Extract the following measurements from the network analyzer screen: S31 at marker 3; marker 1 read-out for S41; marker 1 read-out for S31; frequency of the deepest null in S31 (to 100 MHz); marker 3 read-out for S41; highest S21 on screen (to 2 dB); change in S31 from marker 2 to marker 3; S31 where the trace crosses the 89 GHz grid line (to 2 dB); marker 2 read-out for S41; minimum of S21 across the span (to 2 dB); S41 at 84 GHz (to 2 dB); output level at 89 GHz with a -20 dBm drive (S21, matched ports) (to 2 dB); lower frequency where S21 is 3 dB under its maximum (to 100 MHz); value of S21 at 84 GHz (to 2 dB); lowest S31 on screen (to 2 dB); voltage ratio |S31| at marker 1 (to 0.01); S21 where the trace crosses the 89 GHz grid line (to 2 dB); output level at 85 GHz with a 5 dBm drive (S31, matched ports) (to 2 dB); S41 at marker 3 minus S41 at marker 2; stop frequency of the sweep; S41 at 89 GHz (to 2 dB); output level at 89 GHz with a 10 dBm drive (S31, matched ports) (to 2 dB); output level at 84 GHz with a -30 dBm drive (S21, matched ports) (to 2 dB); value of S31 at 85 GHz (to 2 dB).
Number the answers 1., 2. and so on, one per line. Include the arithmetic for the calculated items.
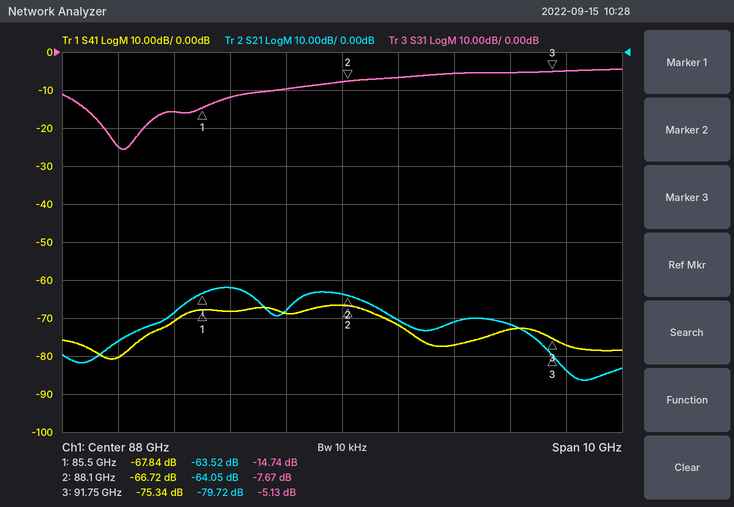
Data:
1. -5.13 dB
2. -67.84 dB
3. -14.74 dB
4. 84.1 GHz
5. -75.34 dB
6. -62 dB
7. -5.13 − (-7.67) = 2.54 dB
8. -6 dB
9. -66.72 dB
10. -86 dB
11. -80 dB
12. -20 dBm + (-70 dB) = -90 dBm
13. 85.3 GHz
14. -76 dB
15. -26 dB
16. 10^(-14.74/20) ≈ 0.18
17. -70 dB
18. 5 dBm + (-16 dB) = -10 dBm
19. -75.34 − (-66.72) = -8.62 dB
20. 93 GHz
21. -72 dB
22. 10 dBm + (-6 dB) = 4 dBm
23. -30 dBm + (-76 dB) = -106 dBm
24. -16 dB
